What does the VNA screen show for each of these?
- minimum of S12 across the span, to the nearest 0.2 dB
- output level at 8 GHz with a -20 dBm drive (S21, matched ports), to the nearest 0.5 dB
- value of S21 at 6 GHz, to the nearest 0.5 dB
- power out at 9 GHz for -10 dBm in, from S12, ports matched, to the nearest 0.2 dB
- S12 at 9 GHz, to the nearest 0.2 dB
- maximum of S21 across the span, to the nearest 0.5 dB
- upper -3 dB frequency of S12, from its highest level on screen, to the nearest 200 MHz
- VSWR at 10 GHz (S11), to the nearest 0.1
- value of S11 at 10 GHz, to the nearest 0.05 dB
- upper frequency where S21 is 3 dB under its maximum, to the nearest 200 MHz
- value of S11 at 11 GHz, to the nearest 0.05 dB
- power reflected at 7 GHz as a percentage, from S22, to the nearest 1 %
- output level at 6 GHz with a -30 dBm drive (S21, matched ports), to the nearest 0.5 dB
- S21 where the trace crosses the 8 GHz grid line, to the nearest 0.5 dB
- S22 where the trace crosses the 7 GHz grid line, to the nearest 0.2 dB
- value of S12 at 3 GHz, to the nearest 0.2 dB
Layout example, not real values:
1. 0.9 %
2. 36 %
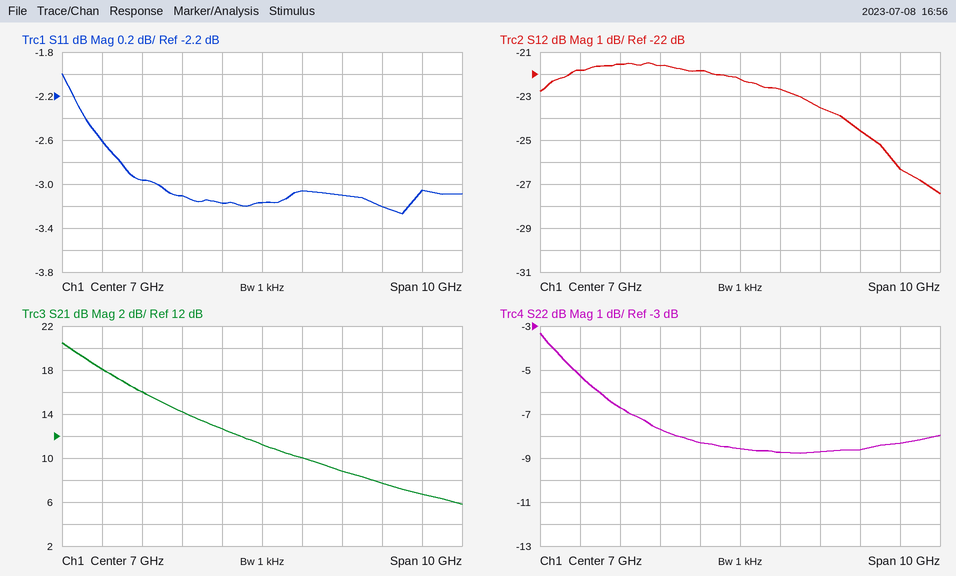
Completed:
1. -27.4 dB
2. -10.0 dBm
3. 12.5 dB
4. -33.6 dBm
5. -23.6 dB
6. 20.5 dB
7. 10.0 GHz
8. 5.5
9. -3.20 dB
10. 3.2 GHz
11. -3.05 dB
12. 14 %
13. -17.5 dBm
14. 10.0 dB
15. -8.6 dB
16. -21.8 dB
